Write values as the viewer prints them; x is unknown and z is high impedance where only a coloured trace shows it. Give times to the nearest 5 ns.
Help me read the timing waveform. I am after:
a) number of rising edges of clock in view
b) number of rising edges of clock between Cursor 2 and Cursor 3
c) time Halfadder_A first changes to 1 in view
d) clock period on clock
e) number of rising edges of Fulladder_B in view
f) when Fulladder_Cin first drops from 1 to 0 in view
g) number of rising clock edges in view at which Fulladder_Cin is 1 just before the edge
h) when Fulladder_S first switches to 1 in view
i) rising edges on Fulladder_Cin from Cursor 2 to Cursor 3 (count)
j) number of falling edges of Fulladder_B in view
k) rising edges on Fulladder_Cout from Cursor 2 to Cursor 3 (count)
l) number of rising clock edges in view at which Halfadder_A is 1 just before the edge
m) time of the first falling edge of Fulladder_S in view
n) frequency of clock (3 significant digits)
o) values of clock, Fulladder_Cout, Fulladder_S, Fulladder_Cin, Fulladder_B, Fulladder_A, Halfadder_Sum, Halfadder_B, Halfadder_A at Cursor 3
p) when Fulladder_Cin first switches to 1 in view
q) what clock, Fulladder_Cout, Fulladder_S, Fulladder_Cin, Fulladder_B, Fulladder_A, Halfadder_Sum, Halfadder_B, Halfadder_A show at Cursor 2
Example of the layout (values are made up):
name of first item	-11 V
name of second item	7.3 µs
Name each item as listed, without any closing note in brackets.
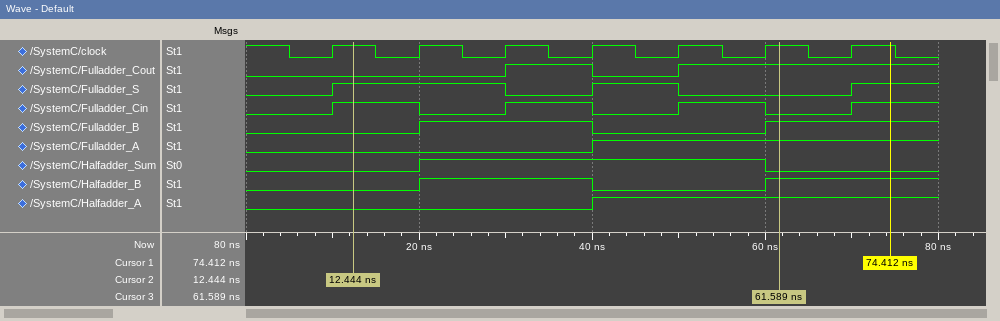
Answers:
number of rising edges of clock in view	7
number of rising edges of clock between Cursor 2 and Cursor 3	5
time Halfadder_A first changes to 1 in view	40 ns
clock period on clock	10 ns
number of rising edges of Fulladder_B in view	2
when Fulladder_Cin first drops from 1 to 0 in view	20 ns
number of rising clock edges in view at which Fulladder_Cin is 1 just before the edge	3
when Fulladder_S first switches to 1 in view	10 ns
rising edges on Fulladder_Cin from Cursor 2 to Cursor 3	2
number of falling edges of Fulladder_B in view	1
rising edges on Fulladder_Cout from Cursor 2 to Cursor 3	2
number of rising clock edges in view at which Halfadder_A is 1 just before the edge	3
time of the first falling edge of Fulladder_S in view	30 ns
frequency of clock	100 MHz
values of clock, Fulladder_Cout, Fulladder_S, Fulladder_Cin, Fulladder_B, Fulladder_A, Halfadder_Sum, Halfadder_B, Halfadder_A at Cursor 3	clock=1, Fulladder_Cout=1, Fulladder_S=0, Fulladder_Cin=0, Fulladder_B=1, Fulladder_A=1, Halfadder_Sum=0, Halfadder_B=1, Halfadder_A=1
when Fulladder_Cin first switches to 1 in view	10 ns
what clock, Fulladder_Cout, Fulladder_S, Fulladder_Cin, Fulladder_B, Fulladder_A, Halfadder_Sum, Halfadder_B, Halfadder_A show at Cursor 2	clock=1, Fulladder_Cout=0, Fulladder_S=1, Fulladder_Cin=1, Fulladder_B=0, Fulladder_A=0, Halfadder_Sum=0, Halfadder_B=0, Halfadder_A=0
